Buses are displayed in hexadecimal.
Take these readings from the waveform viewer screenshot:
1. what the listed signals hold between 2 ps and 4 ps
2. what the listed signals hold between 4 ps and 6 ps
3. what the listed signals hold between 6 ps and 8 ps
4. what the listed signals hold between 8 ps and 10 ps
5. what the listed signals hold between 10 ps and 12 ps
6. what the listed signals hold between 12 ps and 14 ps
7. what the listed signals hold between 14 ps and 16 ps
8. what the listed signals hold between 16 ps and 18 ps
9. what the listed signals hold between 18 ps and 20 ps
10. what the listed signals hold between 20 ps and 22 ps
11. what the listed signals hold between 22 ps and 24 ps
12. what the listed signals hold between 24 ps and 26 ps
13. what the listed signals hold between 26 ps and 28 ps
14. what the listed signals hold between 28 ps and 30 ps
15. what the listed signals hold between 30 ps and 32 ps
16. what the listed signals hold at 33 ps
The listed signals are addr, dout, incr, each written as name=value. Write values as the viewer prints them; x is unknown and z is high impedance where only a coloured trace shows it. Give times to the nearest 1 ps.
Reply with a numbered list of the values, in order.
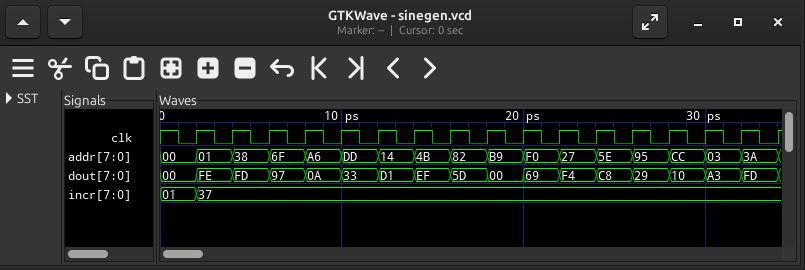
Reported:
1. addr=01, dout=FE, incr=37
2. addr=38, dout=FD, incr=37
3. addr=6F, dout=97, incr=37
4. addr=A6, dout=0A, incr=37
5. addr=DD, dout=33, incr=37
6. addr=14, dout=D1, incr=37
7. addr=4B, dout=EF, incr=37
8. addr=82, dout=5D, incr=37
9. addr=B9, dout=00, incr=37
10. addr=F0, dout=69, incr=37
11. addr=27, dout=F4, incr=37
12. addr=5E, dout=C8, incr=37
13. addr=95, dout=29, incr=37
14. addr=CC, dout=10, incr=37
15. addr=03, dout=A3, incr=37
16. addr=3A, dout=FD, incr=37
